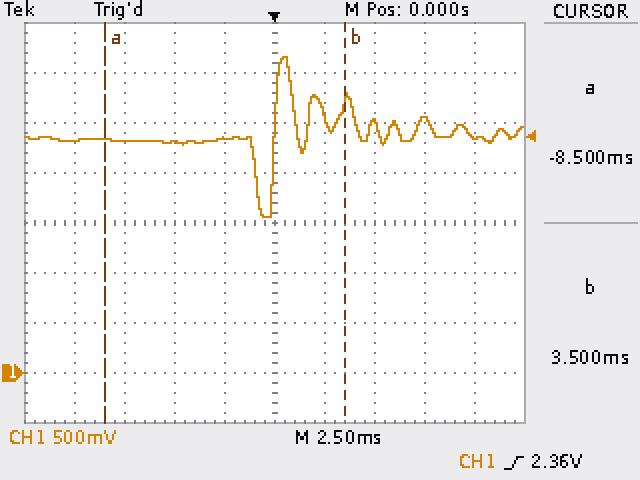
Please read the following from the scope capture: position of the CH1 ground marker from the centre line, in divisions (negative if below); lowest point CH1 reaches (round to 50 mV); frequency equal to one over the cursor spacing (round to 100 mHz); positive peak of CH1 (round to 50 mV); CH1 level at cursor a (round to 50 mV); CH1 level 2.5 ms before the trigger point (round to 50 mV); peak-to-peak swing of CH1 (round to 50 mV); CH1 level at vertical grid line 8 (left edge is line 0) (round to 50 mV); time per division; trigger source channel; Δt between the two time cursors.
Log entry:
-3.0 div
1.55 V
83.3 Hz
3.15 V
2.35 V
2.35 V
1.60 V
2.55 V
2.5 ms
CH1
12.00 ms
